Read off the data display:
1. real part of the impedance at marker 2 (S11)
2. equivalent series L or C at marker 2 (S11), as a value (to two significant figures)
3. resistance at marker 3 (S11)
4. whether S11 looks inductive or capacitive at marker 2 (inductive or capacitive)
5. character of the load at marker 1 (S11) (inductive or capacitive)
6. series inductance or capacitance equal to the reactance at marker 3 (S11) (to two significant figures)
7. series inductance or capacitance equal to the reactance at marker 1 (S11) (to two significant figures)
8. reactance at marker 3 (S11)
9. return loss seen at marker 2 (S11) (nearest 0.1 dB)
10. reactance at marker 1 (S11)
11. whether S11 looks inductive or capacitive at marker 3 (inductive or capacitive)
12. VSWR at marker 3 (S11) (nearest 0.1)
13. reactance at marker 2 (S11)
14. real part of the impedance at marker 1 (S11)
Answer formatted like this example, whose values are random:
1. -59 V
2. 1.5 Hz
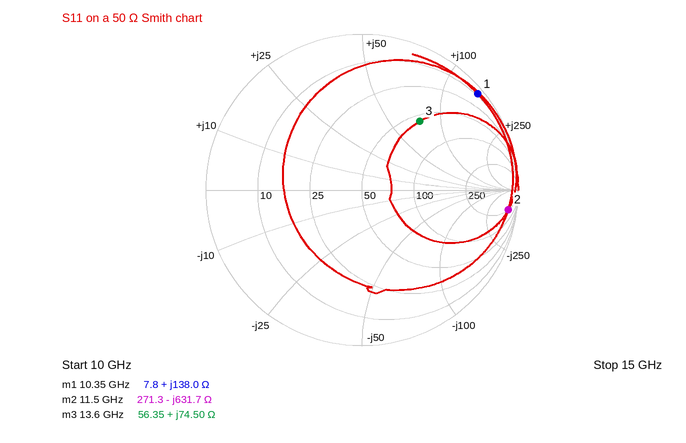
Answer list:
1. 271.3 Ω
2. 22 fF
3. 56.35 Ω
4. capacitive
5. inductive
6. 870 pH
7. 2.1 nH
8. +74.50 Ω
9. 0.5 dB
10. +138.0 Ω
11. inductive
12. 3.7
13. -631.7 Ω
14. 7.8 Ω
